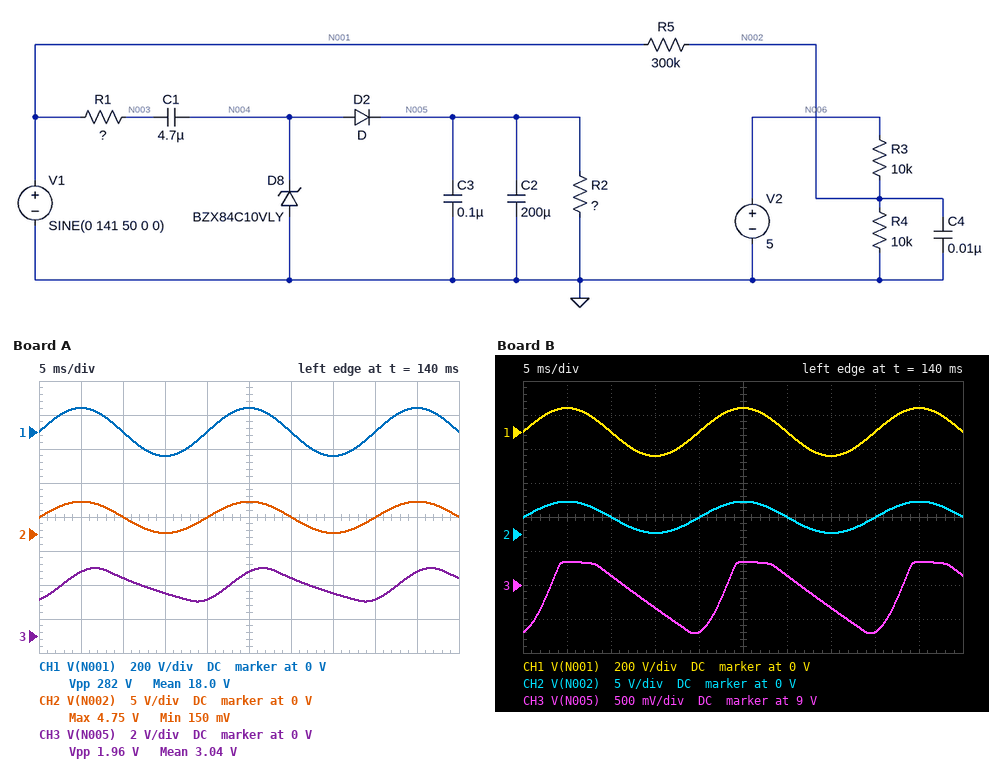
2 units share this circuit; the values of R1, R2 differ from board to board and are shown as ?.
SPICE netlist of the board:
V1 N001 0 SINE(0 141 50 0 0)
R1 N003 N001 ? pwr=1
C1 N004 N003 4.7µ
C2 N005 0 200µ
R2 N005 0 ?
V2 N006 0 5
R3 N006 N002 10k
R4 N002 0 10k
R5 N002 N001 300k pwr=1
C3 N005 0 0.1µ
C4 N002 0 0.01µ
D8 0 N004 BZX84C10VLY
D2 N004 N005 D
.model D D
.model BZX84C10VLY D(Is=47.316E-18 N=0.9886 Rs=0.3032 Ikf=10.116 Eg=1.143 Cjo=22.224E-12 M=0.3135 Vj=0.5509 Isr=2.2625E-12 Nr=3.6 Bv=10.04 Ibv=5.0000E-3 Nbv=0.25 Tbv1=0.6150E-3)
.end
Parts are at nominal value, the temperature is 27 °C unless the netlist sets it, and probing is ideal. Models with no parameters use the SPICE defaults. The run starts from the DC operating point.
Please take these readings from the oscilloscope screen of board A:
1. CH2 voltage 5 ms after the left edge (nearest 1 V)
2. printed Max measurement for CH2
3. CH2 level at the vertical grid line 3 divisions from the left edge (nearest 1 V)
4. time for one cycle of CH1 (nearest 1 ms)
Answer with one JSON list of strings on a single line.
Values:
["5 V", "4.75 V", "0 V", "20 ms"]
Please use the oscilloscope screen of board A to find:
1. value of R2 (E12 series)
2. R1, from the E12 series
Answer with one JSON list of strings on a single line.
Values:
["82 Ω", "1 kΩ"]
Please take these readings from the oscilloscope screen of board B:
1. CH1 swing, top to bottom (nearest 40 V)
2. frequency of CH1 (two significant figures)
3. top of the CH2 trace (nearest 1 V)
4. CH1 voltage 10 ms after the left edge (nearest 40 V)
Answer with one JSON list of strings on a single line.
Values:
["280 V", "50 Hz", "5 V", "0 V"]
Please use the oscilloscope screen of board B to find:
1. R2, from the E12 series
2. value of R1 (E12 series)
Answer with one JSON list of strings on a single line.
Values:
["470 Ω", "1.5 kΩ"]
